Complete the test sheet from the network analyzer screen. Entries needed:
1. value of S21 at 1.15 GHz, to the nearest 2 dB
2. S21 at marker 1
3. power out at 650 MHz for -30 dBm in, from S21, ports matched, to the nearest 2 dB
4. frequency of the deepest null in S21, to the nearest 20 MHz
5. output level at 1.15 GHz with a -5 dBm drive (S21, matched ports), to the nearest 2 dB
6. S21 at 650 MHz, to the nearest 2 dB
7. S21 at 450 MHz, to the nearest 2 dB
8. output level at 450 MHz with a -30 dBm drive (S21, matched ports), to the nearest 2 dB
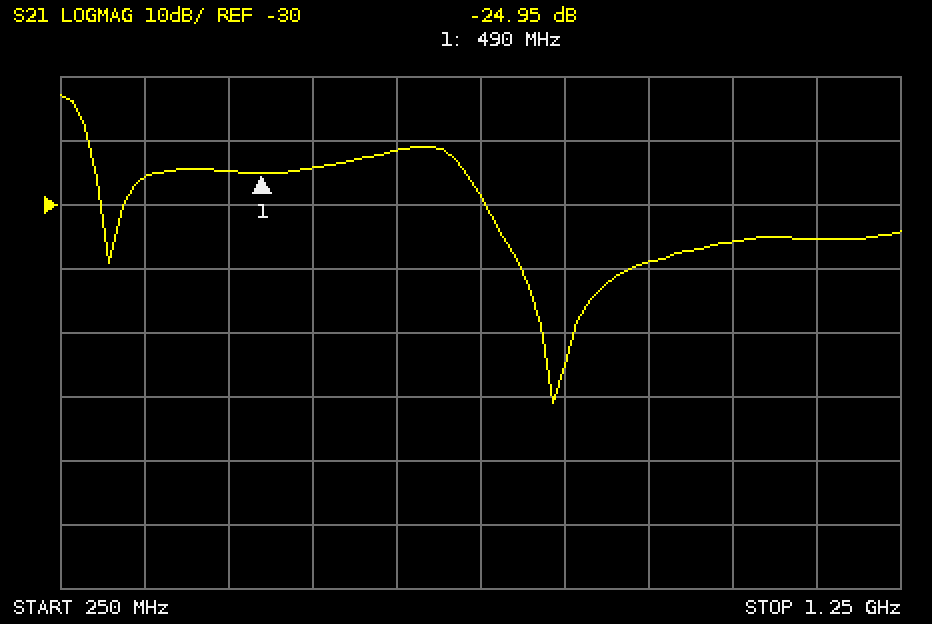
-36 dB
-24.95 dB
-52 dBm
840 MHz
-40 dBm
-22 dB
-24 dB
-54 dBm
